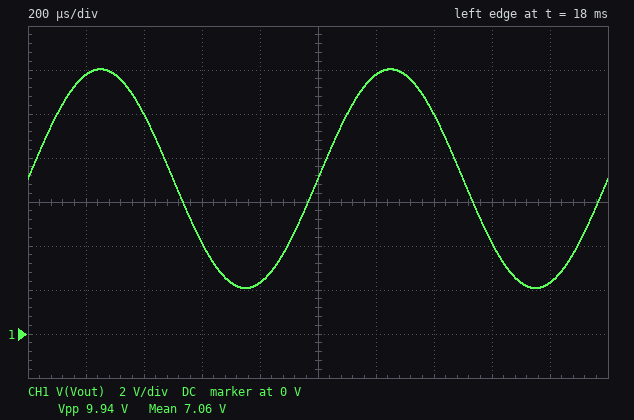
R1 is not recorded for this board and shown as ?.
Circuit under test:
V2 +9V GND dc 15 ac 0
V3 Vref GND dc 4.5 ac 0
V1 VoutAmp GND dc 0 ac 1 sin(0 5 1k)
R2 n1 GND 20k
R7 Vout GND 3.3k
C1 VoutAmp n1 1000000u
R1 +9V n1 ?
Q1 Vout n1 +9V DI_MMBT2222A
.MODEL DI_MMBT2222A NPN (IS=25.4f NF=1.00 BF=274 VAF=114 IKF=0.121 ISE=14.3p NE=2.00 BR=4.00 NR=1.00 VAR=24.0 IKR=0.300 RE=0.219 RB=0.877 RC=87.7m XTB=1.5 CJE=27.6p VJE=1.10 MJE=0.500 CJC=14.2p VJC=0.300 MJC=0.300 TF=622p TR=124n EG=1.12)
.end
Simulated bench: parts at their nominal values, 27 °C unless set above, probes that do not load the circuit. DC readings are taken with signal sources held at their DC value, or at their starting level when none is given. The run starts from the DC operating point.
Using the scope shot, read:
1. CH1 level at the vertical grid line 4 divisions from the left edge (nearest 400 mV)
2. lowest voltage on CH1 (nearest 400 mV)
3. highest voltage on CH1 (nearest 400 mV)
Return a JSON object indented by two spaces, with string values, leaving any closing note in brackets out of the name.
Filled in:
{
  "CH1 level at the vertical grid line 4 divisions from the left edge": "2.4 V",
  "lowest voltage on CH1": "2.0 V",
  "highest voltage on CH1": "12.0 V"
}
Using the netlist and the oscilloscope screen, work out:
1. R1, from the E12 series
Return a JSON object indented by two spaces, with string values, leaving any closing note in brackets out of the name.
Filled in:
{
  "R1, from the E12 series": "10 kΩ"
}
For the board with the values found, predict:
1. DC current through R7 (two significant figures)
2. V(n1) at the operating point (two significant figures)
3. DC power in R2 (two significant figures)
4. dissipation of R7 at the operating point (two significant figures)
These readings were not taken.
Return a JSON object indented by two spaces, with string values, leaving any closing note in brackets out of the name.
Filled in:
{
  "DC current through R7": "2.1 mA",
  "V(n1) at the operating point": "7.7 V",
  "DC power in R2": "3.0 mW",
  "dissipation of R7 at the operating point": "15 mW"
}
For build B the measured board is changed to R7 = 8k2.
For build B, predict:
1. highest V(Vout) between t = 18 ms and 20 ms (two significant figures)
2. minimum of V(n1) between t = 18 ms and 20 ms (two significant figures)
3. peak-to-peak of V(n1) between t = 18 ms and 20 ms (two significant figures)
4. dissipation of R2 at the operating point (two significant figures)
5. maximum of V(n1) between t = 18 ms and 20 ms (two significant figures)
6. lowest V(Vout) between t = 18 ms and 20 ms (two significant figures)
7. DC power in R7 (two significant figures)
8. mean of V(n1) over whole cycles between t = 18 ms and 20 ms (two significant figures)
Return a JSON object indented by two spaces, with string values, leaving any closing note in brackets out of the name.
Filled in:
{
  "highest V(Vout) between t = 18 ms and 20 ms": "13 V",
  "minimum of V(n1) between t = 18 ms and 20 ms": "3.9 V",
  "peak-to-peak of V(n1) between t = 18 ms and 20 ms": "10 V",
  "dissipation of R2 at the operating point": "3.9 mW",
  "maximum of V(n1) between t = 18 ms and 20 ms": "14 V",
  "lowest V(Vout) between t = 18 ms and 20 ms": "3.3 V",
  "DC power in R7": "8.3 mW",
  "mean of V(n1) over whole cycles between t = 18 ms and 20 ms": "8.9 V"
}
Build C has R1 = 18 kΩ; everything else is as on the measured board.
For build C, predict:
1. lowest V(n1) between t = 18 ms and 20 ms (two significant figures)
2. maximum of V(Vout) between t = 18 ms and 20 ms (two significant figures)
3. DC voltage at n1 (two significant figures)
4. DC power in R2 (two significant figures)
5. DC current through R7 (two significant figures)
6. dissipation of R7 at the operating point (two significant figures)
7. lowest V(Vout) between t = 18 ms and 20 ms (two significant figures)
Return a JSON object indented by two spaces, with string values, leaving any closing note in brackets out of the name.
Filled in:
{
  "lowest V(n1) between t = 18 ms and 20 ms": "670 mV",
  "maximum of V(Vout) between t = 18 ms and 20 ms": "10 V",
  "DC voltage at n1": "5.7 V",
  "DC power in R2": "1.6 mW",
  "DC current through R7": "1.5 mA",
  "dissipation of R7 at the operating point": "7.7 mW",
  "lowest V(Vout) between t = 18 ms and 20 ms": "140 mV"
}
